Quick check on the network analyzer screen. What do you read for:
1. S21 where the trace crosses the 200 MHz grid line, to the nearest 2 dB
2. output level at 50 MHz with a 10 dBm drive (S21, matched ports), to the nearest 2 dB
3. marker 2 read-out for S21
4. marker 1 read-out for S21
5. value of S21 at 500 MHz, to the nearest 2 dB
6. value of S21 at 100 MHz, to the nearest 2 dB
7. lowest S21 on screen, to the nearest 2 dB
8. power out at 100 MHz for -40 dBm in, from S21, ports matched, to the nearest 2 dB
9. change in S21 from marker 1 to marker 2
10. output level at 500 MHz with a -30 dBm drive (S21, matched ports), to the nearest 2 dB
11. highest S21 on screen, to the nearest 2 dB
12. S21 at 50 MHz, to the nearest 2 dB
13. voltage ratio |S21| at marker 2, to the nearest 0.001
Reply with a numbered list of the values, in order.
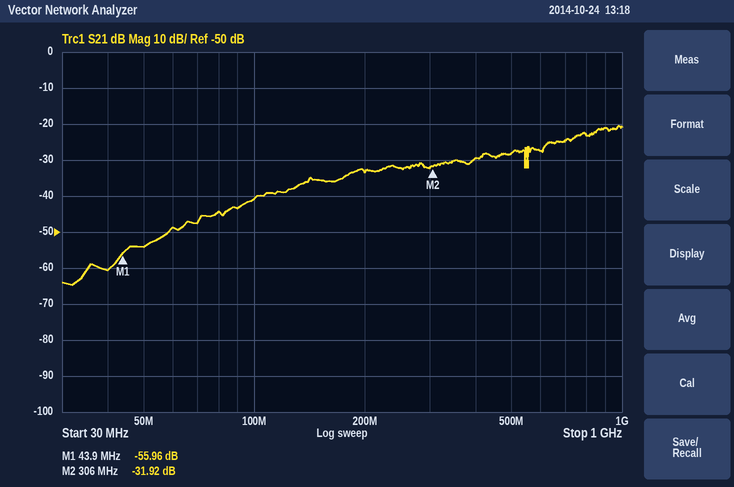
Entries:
1. -34 dB
2. -44 dBm
3. -31.92 dB
4. -55.96 dB
5. -28 dB
6. -40 dB
7. -64 dB
8. -80 dBm
9. 24.04 dB
10. -58 dBm
11. -20 dB
12. -54 dB
13. 0.025
